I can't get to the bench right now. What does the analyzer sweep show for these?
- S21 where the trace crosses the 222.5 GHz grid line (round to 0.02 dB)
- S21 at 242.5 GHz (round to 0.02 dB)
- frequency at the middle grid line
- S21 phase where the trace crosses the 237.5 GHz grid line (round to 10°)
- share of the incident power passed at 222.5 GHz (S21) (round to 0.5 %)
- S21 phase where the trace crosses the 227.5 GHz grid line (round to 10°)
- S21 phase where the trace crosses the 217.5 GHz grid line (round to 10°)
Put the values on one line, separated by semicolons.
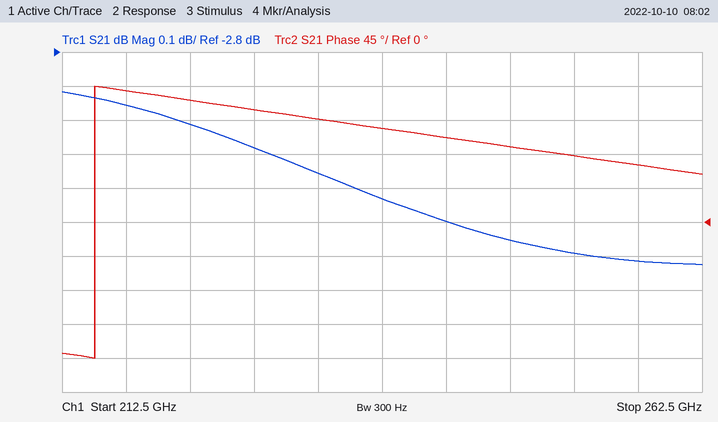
-3.02 dB; -3.30 dB; 237.5 GHz; 120°; 50.0 %; 150°; 170°
